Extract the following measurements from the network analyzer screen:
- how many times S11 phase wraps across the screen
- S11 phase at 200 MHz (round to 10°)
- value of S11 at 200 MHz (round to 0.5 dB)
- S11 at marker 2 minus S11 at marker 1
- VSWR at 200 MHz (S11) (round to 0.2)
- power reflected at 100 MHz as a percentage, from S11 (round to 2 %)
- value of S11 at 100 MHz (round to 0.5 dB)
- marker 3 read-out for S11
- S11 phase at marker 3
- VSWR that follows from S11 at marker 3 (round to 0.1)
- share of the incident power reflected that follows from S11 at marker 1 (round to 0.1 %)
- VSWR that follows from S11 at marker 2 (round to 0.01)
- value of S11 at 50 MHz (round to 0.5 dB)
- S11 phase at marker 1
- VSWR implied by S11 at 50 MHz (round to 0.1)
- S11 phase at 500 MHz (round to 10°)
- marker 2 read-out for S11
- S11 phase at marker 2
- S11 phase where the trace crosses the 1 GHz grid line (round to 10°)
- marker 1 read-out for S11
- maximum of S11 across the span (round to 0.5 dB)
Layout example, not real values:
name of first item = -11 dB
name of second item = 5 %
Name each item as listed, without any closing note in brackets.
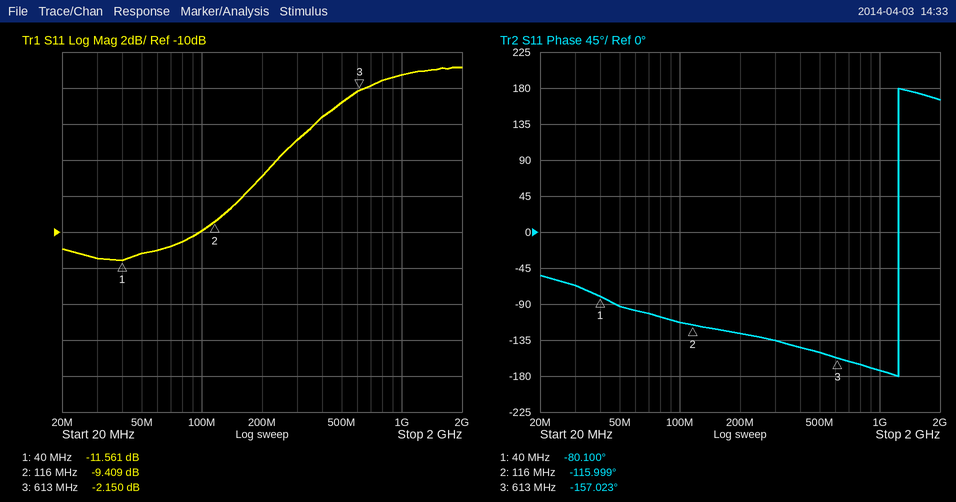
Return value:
how many times S11 phase wraps across the screen = 1
S11 phase at 200 MHz = -130°
value of S11 at 200 MHz = -7.0 dB
S11 at marker 2 minus S11 at marker 1 = 2.152 dB
VSWR at 200 MHz (S11) = 2.6
power reflected at 100 MHz as a percentage, from S11 = 10 %
value of S11 at 100 MHz = -10.0 dB
marker 3 read-out for S11 = -2.150 dB
S11 phase at marker 3 = -157.023°
VSWR that follows from S11 at marker 3 = 8.1
share of the incident power reflected that follows from S11 at marker 1 = 7.0 %
VSWR that follows from S11 at marker 2 = 2.02
value of S11 at 50 MHz = -11.0 dB
S11 phase at marker 1 = -80.100°
VSWR implied by S11 at 50 MHz = 1.8
S11 phase at 500 MHz = -150°
marker 2 read-out for S11 = -9.409 dB
S11 phase at marker 2 = -115.999°
S11 phase where the trace crosses the 1 GHz grid line = -170°
marker 1 read-out for S11 = -11.561 dB
maximum of S11 across the span = -1.0 dB
